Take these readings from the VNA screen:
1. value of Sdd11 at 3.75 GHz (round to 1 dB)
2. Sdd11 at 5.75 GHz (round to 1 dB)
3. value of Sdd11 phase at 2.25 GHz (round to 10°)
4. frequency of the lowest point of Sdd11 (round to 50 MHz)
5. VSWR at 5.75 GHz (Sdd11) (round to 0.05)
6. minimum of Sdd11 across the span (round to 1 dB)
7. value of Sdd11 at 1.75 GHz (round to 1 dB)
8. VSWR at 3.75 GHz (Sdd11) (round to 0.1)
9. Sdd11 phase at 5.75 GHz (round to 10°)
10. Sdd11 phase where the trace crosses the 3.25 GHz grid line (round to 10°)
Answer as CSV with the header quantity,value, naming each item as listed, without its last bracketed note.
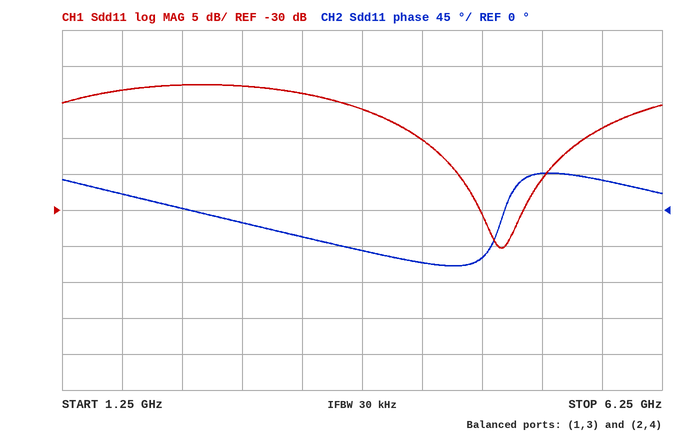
quantity,value
value of Sdd11 at 3.75 GHz,-16 dB
Sdd11 at 5.75 GHz,-19 dB
value of Sdd11 phase at 2.25 GHz,0°
frequency of the lowest point of Sdd11,4.90 GHz
VSWR at 5.75 GHz (Sdd11),1.25
minimum of Sdd11 across the span,-35 dB
value of Sdd11 at 1.75 GHz,-13 dB
VSWR at 3.75 GHz (Sdd11),1.4
Sdd11 phase at 5.75 GHz,40°
Sdd11 phase where the trace crosses the 3.25 GHz grid line,-30°
